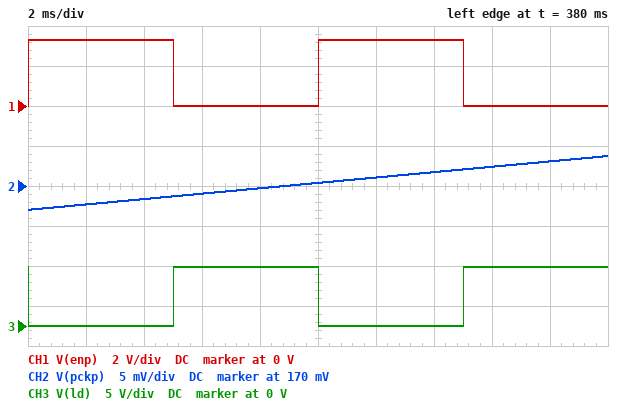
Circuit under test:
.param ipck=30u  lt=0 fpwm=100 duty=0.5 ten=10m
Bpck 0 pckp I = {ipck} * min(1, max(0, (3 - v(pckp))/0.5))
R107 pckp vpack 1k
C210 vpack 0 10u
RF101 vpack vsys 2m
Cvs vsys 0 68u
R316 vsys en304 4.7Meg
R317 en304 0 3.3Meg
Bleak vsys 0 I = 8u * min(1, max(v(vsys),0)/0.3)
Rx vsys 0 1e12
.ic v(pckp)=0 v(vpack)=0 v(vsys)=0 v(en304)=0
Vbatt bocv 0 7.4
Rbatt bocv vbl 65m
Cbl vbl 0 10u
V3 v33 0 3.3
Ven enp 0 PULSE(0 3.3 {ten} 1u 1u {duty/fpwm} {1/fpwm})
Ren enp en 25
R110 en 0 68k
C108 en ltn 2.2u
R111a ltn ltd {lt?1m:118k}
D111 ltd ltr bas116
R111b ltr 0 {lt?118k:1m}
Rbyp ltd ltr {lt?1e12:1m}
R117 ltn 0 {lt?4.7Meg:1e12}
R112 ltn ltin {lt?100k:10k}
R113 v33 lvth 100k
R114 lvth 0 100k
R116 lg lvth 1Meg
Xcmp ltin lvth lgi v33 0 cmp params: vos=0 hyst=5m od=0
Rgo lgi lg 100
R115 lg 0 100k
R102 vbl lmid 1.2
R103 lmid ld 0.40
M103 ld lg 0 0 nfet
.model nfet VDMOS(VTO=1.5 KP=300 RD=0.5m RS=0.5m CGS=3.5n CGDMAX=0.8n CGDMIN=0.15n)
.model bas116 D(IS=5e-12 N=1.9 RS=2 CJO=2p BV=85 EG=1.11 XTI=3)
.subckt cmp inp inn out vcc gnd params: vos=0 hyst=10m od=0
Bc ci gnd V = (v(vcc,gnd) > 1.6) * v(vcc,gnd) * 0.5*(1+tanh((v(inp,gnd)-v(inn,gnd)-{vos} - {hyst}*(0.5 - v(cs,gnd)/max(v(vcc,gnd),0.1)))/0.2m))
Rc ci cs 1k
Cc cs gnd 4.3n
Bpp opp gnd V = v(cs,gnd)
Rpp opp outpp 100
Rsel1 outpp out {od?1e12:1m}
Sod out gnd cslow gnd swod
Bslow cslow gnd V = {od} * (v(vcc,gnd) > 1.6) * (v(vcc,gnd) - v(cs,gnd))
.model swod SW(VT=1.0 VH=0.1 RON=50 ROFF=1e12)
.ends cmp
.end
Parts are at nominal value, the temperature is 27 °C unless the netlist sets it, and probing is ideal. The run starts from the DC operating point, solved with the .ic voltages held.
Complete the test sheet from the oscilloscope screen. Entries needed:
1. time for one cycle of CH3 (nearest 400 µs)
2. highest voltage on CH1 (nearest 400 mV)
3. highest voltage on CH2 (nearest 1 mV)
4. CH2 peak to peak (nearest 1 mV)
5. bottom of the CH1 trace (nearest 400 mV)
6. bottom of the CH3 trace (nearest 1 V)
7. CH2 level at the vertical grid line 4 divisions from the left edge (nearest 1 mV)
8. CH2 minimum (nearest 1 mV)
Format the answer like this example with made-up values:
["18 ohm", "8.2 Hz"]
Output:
["10.0 ms", "3.2 V", "174 mV", "7 mV", "0 V", "0 V", "170 mV", "167 mV"]
